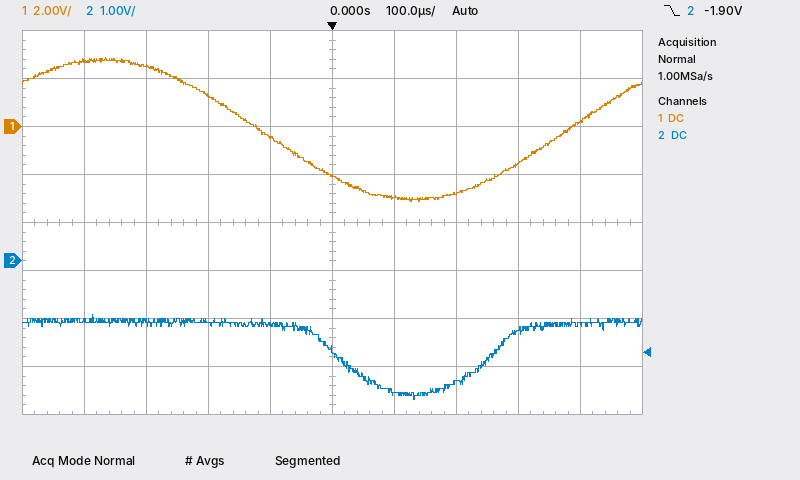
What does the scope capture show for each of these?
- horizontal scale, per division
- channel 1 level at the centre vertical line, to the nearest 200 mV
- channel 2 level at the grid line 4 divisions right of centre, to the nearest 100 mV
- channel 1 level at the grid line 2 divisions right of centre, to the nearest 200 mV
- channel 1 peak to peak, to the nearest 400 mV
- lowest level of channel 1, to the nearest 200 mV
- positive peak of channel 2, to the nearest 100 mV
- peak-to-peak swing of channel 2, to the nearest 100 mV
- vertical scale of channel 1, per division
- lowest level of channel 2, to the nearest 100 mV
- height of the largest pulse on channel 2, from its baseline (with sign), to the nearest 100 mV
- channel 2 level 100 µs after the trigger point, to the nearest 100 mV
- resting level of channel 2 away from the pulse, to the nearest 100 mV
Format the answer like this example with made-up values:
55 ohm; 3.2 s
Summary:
100 µs; -2.0 V; -1.3 V; -2.8 V; 6.0 V; -3.2 V; -1.1 V; 1.8 V; 2 V; -2.9 V; -1.6 V; -2.7 V; -1.3 V
